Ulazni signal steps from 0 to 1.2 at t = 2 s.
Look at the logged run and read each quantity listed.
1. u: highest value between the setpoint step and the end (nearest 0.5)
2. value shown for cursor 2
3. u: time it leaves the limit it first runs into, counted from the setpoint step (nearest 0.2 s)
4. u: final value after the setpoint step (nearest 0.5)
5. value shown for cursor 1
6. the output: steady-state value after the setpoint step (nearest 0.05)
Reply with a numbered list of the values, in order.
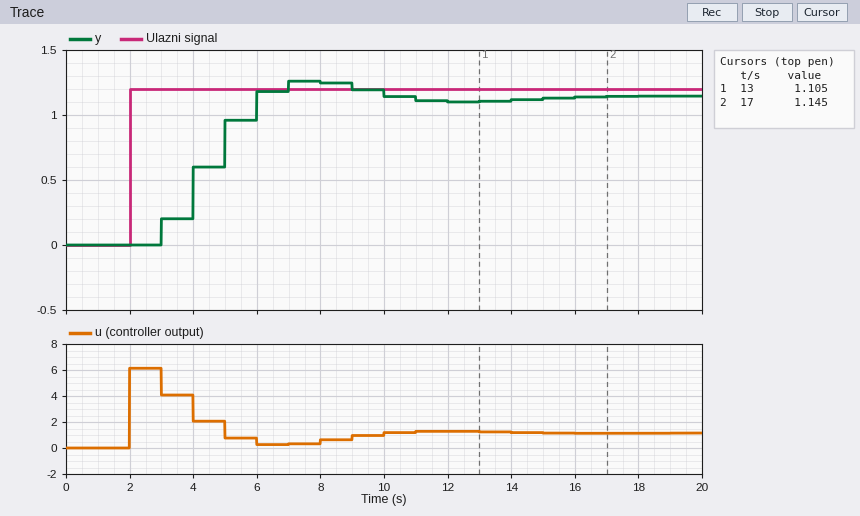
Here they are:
1. 6.0
2. 1.145
3. 1.0 s
4. 1.0
5. 1.105
6. 1.15
